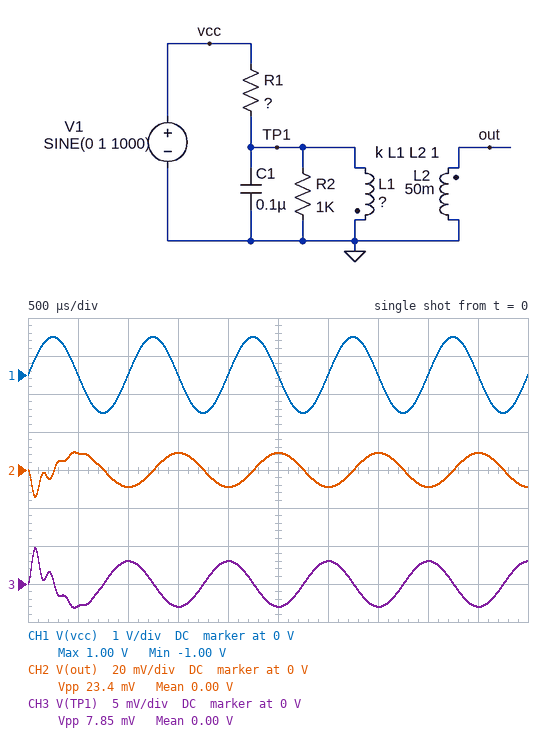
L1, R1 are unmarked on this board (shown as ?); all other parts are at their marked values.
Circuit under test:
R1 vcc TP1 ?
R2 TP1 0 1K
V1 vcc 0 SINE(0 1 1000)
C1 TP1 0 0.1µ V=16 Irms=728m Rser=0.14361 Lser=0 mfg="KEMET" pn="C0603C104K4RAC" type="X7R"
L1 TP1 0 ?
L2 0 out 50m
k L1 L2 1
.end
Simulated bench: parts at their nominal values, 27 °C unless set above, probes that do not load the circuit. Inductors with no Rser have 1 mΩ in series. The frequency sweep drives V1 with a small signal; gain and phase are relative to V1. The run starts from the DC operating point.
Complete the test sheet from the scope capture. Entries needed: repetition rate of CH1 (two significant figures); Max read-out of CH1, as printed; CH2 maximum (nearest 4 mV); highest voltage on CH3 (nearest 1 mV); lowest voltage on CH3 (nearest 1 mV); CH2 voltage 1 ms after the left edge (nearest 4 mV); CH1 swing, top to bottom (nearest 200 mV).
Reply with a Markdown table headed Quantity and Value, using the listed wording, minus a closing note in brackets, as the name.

| Quantity | Value |
|---|---|
| repetition rate of CH1 | 1.0 kHz |
| Max read-out of CH1, as printed | 1.00 V |
| CH2 maximum | 8 mV |
| highest voltage on CH3 | 5 mV |
| lowest voltage on CH3 | -3 mV |
| CH2 voltage 1 ms after the left edge | -8 mV |
| CH1 swing, top to bottom | 2.0 V |
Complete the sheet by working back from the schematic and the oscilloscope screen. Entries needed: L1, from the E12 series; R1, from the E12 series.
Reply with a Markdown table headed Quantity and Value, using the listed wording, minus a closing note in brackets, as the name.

| Quantity | Value |
|---|---|
| L1, from the E12 series | 5.6 mH |
| R1, from the E12 series | 12 kΩ |
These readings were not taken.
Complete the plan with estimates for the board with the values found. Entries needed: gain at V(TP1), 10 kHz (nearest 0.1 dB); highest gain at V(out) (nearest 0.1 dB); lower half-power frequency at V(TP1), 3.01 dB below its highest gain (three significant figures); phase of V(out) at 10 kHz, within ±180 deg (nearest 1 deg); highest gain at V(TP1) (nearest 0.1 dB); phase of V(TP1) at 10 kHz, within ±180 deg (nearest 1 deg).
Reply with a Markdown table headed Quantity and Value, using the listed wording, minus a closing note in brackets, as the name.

| Quantity | Value |
|---|---|
| gain at V(TP1), 10 kHz | -32.7 dB |
| highest gain at V(out) | -12.8 dB |
| lower half-power frequency at V(TP1), 3.01 dB below its highest gain | 5.92 kHz |
| phase of V(out) at 10 kHz, within ±180 deg | 108 deg |
| highest gain at V(TP1) | -22.3 dB |
| phase of V(TP1) at 10 kHz, within ±180 deg | -72 deg |
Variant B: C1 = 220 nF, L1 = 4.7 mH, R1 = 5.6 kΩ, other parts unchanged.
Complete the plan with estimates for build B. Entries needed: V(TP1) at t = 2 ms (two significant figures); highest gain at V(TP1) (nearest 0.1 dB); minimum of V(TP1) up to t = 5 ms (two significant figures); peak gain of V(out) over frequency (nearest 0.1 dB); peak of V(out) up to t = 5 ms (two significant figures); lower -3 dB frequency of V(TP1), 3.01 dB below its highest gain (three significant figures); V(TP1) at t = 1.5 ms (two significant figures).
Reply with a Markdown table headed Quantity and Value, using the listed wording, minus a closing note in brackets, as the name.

| Quantity | Value |
|---|---|
| V(TP1) at t = 2 ms | 5.5 mV |
| highest gain at V(TP1) | -16.4 dB |
| minimum of V(TP1) up to t = 5 ms | -6.4 mV |
| peak gain of V(out) over frequency | -6.2 dB |
| peak of V(out) up to t = 5 ms | 21 mV |
| lower -3 dB frequency of V(TP1), 3.01 dB below its highest gain | 4.54 kHz |
| V(TP1) at t = 1.5 ms | -5.4 mV |
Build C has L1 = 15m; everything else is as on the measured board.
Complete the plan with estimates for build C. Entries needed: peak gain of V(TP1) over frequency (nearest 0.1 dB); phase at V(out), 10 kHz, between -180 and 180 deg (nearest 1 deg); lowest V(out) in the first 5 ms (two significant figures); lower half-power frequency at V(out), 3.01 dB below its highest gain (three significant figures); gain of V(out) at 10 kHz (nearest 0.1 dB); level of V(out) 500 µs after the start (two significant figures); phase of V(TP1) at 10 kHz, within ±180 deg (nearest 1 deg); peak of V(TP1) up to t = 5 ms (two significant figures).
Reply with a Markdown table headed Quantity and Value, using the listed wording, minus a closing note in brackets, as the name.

| Quantity | Value |
|---|---|
| peak gain of V(TP1) over frequency | -22.3 dB |
| phase at V(out), 10 kHz, between -180 and 180 deg | 102 deg |
| lowest V(out) in the first 5 ms | -20 mV |
| lower half-power frequency at V(out), 3.01 dB below its highest gain | 3.34 kHz |
| gain of V(out) at 10 kHz | -30.9 dB |
| level of V(out) 500 µs after the start | 16 mV |
| phase of V(TP1) at 10 kHz, within ±180 deg | -78 deg |
| peak of V(TP1) up to t = 5 ms | 11 mV |
